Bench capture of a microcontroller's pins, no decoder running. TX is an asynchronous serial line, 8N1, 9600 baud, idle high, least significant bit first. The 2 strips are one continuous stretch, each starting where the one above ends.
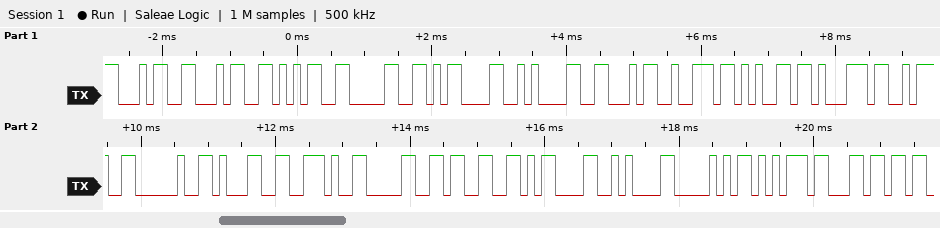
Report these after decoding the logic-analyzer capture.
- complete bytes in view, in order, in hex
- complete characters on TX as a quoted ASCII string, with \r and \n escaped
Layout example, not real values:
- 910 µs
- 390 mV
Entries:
- 34 34 35 30 0D 0A 46 72 65 71 3A 20 31 2E 30 33 0D 0A 50 75 6C
- "4450\r\nFreq: 1.03\r\nPul"
